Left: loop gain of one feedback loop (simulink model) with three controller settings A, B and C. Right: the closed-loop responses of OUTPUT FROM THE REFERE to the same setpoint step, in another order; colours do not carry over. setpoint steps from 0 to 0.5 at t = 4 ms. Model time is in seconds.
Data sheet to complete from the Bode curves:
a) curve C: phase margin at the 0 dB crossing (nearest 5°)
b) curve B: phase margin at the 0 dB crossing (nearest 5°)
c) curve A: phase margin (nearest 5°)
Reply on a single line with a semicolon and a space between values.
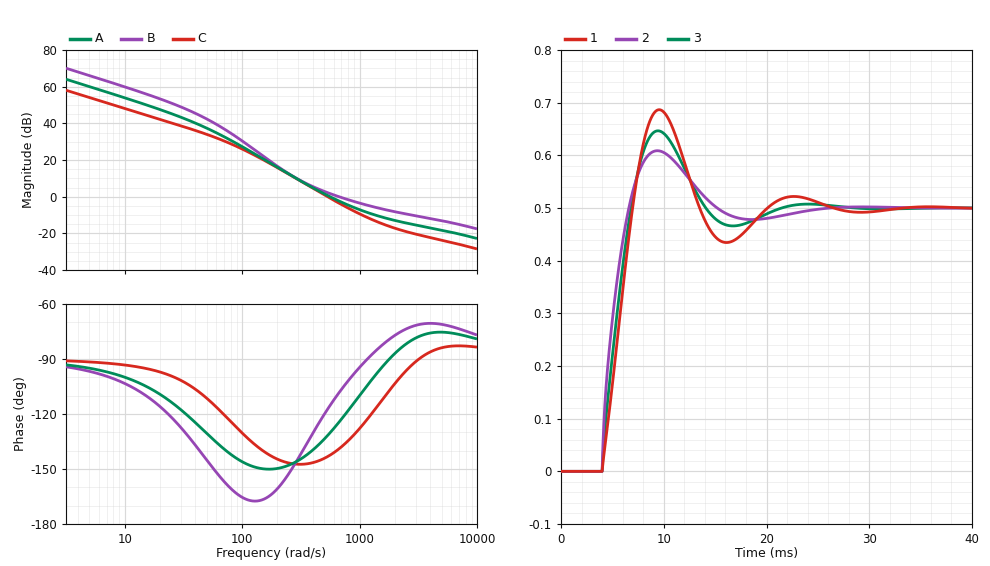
35°; 70°; 50°
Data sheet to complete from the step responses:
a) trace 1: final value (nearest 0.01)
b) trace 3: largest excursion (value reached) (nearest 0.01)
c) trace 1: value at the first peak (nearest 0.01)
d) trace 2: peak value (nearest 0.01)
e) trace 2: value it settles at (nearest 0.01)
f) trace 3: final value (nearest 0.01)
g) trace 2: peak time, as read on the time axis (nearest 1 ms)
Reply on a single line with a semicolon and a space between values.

0.50; 0.65; 0.69; 0.61; 0.50; 0.50; 9 ms
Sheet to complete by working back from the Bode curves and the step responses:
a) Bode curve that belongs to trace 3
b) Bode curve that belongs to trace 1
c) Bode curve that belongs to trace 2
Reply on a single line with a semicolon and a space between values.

A; C; B
